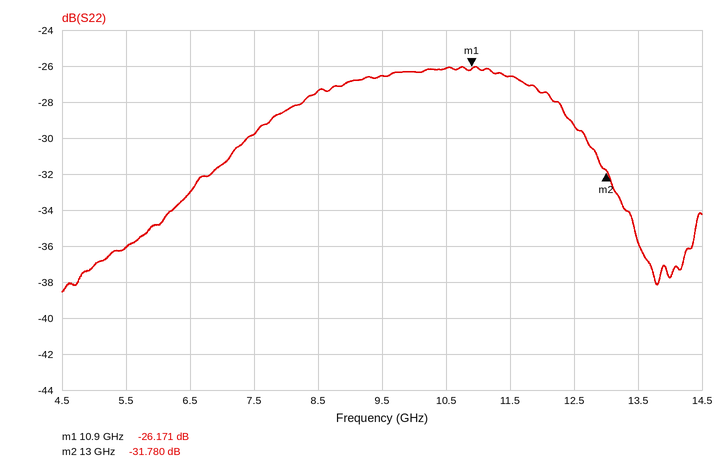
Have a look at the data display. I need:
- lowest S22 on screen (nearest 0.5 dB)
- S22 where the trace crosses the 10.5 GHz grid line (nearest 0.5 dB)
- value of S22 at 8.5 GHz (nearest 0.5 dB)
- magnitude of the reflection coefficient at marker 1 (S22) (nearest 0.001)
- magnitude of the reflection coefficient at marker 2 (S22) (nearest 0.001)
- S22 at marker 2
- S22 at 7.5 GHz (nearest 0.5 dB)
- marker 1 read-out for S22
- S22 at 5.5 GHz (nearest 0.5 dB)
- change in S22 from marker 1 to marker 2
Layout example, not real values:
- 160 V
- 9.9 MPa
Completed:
- -38.5 dB
- -26.0 dB
- -27.5 dB
- 0.049
- 0.026
- -31.780 dB
- -30.0 dB
- -26.171 dB
- -36.0 dB
- -5.609 dB
